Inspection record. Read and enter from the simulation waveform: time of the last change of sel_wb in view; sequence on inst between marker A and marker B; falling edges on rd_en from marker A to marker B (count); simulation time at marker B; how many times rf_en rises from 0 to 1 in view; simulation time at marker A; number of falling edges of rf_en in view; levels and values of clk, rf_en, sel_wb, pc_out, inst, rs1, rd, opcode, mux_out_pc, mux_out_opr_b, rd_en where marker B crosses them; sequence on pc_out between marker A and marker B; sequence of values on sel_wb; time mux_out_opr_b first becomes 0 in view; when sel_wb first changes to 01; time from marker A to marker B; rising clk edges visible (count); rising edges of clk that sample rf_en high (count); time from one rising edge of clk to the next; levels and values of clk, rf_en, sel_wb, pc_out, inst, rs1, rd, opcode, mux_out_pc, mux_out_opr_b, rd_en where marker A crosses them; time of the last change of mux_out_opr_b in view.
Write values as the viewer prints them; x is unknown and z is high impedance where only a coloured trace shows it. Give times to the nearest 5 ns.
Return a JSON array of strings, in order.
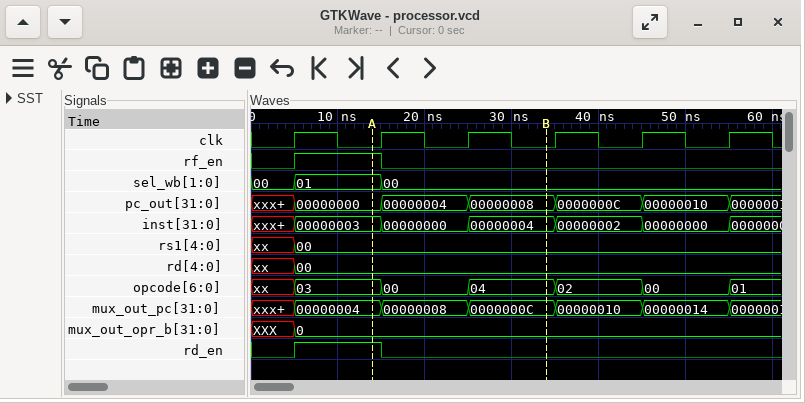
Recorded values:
["15 ns", "00000003, 00000000, 00000004", "1", "35 ns", "1", "15 ns", "1", "clk=0, rf_en=0, sel_wb=00, pc_out=00000008, inst=00000004, rs1=00, rd=00, opcode=04, mux_out_pc=0000000C, mux_out_opr_b=0, rd_en=0", "00000000, 00000004, 00000008", "00, 01, 00", "5 ns", "5 ns", "20 ns", "6", "1", "10 ns", "clk=0, rf_en=1, sel_wb=01, pc_out=00000000, inst=00000003, rs1=00, rd=00, opcode=03, mux_out_pc=00000004, mux_out_opr_b=0, rd_en=1", "5 ns"]
